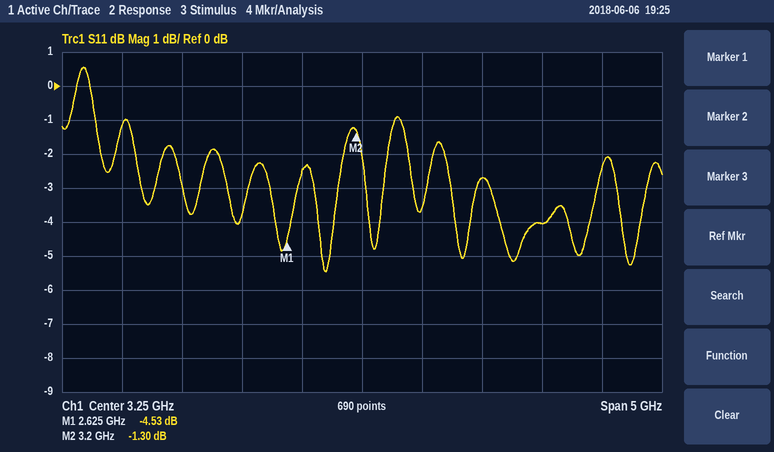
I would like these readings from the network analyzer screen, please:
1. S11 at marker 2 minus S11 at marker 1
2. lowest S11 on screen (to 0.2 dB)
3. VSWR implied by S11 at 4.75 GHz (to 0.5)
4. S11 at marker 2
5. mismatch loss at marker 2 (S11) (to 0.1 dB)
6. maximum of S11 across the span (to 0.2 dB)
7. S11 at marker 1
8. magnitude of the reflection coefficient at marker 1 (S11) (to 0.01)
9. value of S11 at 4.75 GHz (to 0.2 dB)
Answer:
3.23 dB
-5.4 dB
4.5
-1.30 dB
5.9 dB
0.6 dB
-4.53 dB
0.59
-4.0 dB
